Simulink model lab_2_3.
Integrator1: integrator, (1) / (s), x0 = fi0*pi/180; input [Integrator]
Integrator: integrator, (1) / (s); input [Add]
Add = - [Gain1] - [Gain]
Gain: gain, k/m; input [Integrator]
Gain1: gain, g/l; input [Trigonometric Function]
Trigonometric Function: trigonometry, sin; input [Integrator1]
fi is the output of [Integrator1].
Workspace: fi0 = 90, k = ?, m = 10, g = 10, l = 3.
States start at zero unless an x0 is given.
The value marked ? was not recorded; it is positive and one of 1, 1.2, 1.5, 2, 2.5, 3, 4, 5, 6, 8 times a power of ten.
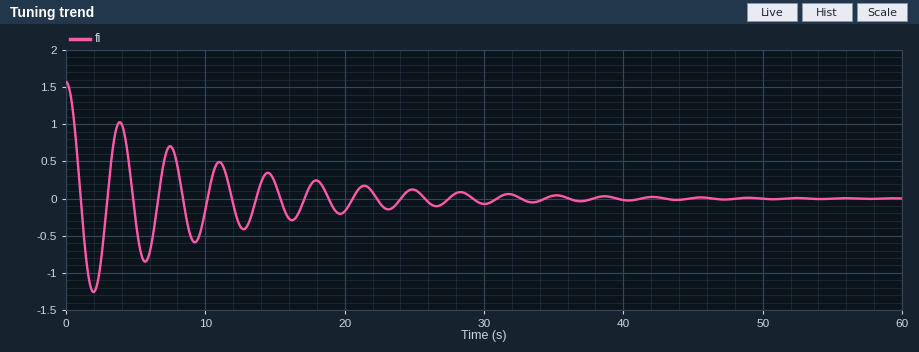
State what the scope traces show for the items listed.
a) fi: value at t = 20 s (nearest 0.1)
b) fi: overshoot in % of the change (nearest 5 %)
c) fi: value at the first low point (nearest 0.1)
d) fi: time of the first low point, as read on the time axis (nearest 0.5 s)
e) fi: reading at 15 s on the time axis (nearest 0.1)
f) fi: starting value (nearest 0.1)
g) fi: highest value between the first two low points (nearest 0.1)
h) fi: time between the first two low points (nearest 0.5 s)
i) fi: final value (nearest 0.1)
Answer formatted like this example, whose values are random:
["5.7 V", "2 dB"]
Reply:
["-0.2", "80 %", "-1.3", "2.0 s", "0.2", "1.6", "1.0", "3.5 s", "0.0"]
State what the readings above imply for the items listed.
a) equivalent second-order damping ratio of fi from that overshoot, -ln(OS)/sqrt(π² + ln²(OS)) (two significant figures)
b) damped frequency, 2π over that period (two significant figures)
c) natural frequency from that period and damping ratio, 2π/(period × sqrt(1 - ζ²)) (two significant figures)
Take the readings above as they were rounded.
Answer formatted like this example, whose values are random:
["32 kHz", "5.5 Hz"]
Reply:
["0.071", "1.8 rad/s", "1.8 rad/s"]
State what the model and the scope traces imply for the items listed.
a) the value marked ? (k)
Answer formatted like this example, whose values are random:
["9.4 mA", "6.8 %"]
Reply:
["2"]
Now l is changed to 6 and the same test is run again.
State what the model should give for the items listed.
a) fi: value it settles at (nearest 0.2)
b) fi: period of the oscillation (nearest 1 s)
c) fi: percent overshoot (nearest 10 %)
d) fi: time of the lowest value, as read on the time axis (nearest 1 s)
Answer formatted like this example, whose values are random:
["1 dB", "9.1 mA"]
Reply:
["0.0", "5 s", "70 %", "3 s"]
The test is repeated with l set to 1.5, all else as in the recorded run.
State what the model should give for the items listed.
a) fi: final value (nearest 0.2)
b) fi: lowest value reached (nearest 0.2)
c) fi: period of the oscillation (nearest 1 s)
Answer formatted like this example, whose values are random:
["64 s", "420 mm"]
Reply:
["0.0", "-1.4", "3 s"]
